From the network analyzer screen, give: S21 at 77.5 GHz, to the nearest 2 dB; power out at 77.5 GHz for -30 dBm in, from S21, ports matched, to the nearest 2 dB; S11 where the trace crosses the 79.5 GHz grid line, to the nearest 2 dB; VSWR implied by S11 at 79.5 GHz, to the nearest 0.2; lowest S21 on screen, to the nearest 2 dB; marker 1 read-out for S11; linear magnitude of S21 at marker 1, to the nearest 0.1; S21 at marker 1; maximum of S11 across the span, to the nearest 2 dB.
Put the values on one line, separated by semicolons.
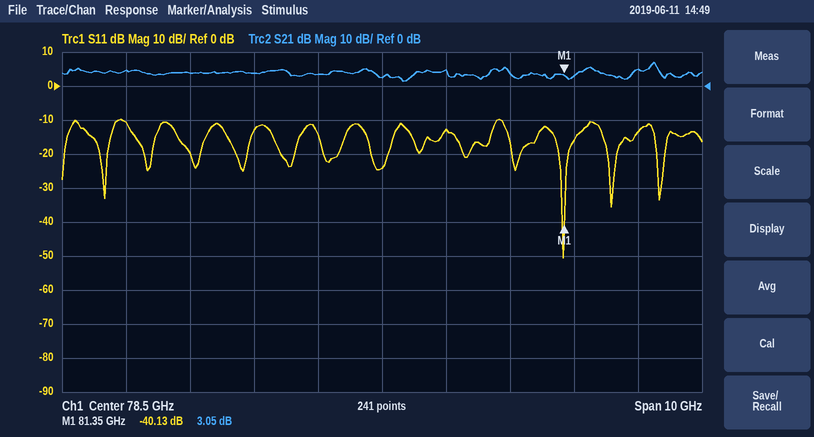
4 dB; -26 dBm; -12 dB; 1.6; 2 dB; -40.13 dB; 1.4; 3.05 dB; -10 dB
